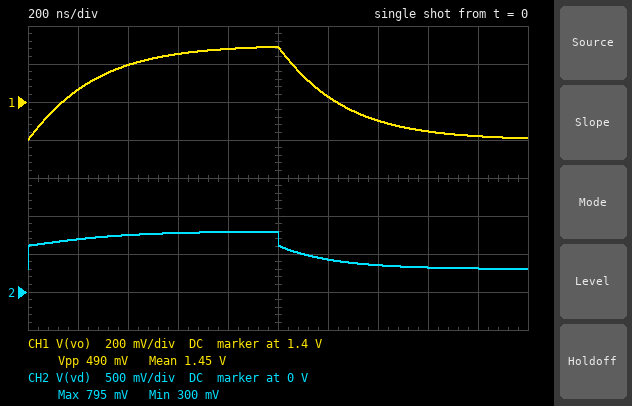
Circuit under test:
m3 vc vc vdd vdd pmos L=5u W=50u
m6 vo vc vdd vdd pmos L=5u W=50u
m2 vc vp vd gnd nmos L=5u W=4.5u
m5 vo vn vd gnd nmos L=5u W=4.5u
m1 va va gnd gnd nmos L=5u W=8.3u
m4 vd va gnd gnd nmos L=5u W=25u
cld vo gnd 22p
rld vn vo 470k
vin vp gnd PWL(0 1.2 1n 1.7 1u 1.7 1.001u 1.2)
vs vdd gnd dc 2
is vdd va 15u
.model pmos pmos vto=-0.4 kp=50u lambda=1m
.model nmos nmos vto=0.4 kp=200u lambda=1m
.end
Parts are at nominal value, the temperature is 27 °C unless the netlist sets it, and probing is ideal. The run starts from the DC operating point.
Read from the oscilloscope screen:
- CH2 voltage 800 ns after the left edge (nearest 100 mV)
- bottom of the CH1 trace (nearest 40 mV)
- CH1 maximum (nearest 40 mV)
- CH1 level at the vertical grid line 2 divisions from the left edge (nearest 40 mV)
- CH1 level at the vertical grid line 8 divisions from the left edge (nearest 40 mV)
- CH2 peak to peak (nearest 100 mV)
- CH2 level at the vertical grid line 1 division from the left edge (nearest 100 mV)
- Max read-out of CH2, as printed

800 mV
1.20 V
1.68 V
1.60 V
1.24 V
500 mV
700 mV
795 mV
